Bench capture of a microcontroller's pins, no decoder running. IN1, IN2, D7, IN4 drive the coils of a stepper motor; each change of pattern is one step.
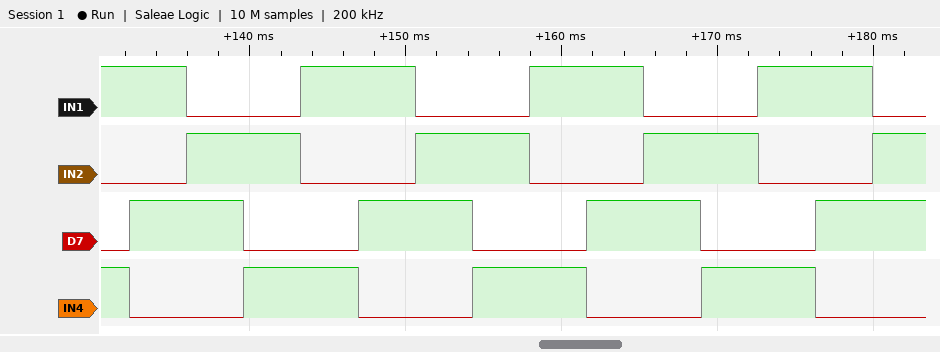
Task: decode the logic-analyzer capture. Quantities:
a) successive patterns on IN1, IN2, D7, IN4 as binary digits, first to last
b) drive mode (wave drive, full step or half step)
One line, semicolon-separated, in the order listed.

1001 1010 0110 0101 1001 1010 0110 0101 1001 1010 0110 0101 1001 1010 0110; full step
